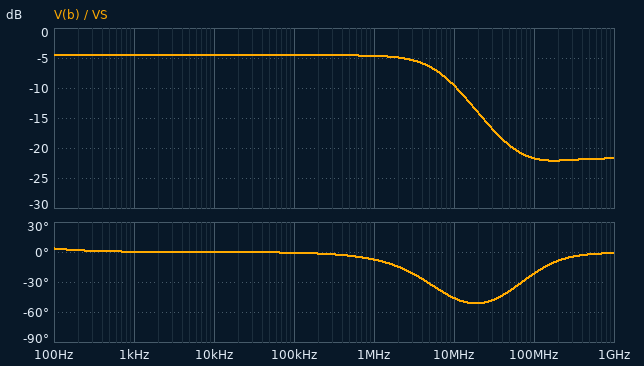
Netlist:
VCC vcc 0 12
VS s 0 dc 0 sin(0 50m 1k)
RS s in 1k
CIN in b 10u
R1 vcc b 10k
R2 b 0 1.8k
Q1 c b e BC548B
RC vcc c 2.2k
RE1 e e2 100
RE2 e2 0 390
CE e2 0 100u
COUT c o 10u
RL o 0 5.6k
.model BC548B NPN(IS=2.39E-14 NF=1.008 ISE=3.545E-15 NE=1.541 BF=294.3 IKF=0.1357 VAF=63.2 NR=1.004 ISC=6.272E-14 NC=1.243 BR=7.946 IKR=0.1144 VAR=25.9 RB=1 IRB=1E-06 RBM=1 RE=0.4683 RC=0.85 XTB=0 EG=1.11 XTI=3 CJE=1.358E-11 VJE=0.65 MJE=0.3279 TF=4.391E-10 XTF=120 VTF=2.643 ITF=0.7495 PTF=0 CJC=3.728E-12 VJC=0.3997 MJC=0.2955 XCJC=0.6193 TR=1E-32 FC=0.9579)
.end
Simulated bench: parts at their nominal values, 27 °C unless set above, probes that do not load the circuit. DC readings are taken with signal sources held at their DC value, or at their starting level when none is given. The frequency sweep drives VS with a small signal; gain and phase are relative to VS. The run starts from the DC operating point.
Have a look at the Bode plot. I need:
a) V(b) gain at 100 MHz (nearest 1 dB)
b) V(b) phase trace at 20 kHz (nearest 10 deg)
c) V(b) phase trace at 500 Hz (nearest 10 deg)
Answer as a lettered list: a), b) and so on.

a) -22 dB
b) 0 deg
c) 0 deg
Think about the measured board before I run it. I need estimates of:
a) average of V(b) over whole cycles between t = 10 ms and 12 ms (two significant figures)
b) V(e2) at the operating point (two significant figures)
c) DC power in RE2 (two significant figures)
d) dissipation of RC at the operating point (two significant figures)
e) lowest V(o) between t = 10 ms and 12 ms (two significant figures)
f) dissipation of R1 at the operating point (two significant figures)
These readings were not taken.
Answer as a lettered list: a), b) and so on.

a) 1.8 V
b) 920 mV
c) 2.2 mW
d) 12 mW
e) -410 mV
f) 10 mW
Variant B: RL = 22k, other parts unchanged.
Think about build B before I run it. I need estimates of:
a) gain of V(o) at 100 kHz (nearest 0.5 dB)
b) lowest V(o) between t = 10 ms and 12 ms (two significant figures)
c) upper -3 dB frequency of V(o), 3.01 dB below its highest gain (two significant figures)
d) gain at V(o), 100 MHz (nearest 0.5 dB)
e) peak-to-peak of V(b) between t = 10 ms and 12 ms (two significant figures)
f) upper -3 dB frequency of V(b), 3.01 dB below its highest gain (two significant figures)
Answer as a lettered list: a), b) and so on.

a) 20.5 dB
b) -520 mV
c) 5.6 MHz
d) -5.0 dB
e) 59 mV
f) 5.7 MHz
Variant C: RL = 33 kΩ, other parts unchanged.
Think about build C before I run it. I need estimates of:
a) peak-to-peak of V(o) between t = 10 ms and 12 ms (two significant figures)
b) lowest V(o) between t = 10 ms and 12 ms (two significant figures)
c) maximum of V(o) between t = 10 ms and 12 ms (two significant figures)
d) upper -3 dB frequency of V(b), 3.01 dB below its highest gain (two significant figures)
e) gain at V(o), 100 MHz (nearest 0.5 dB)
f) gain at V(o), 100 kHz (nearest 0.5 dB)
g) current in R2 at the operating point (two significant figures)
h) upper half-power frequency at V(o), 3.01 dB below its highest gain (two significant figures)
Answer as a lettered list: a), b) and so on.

a) 1.1 V
b) -540 mV
c) 540 mV
d) 5.5 MHz
e) -5.0 dB
f) 20.5 dB
g) 1.0 mA
h) 5.4 MHz
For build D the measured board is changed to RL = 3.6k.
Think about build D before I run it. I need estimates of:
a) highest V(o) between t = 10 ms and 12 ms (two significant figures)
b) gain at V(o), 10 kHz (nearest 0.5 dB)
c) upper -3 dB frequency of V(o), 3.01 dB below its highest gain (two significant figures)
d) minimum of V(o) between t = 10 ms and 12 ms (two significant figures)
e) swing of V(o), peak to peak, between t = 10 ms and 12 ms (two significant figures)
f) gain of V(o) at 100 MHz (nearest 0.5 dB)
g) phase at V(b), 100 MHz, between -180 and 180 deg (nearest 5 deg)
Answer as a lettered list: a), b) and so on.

a) 360 mV
b) 17.0 dB
c) 7.3 MHz
d) -360 mV
e) 720 mV
f) -6.0 dB
g) -25 deg
